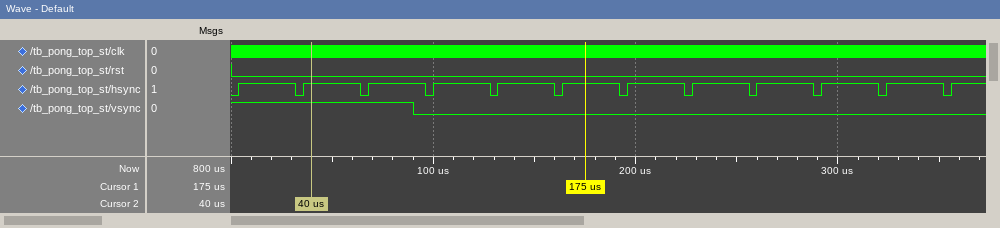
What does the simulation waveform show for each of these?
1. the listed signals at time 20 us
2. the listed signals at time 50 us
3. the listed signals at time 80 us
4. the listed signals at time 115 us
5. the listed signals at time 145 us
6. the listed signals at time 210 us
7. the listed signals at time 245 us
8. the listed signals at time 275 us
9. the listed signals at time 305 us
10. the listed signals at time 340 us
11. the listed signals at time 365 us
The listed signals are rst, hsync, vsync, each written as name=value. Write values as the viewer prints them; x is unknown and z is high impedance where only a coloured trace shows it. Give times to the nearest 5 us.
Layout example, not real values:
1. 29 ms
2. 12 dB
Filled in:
1. rst=0, hsync=1, vsync=1
2. rst=0, hsync=1, vsync=1
3. rst=0, hsync=1, vsync=1
4. rst=0, hsync=1, vsync=0
5. rst=0, hsync=1, vsync=0
6. rst=0, hsync=1, vsync=0
7. rst=0, hsync=1, vsync=0
8. rst=0, hsync=1, vsync=0
9. rst=0, hsync=1, vsync=0
10. rst=0, hsync=1, vsync=0
11. rst=0, hsync=1, vsync=0
